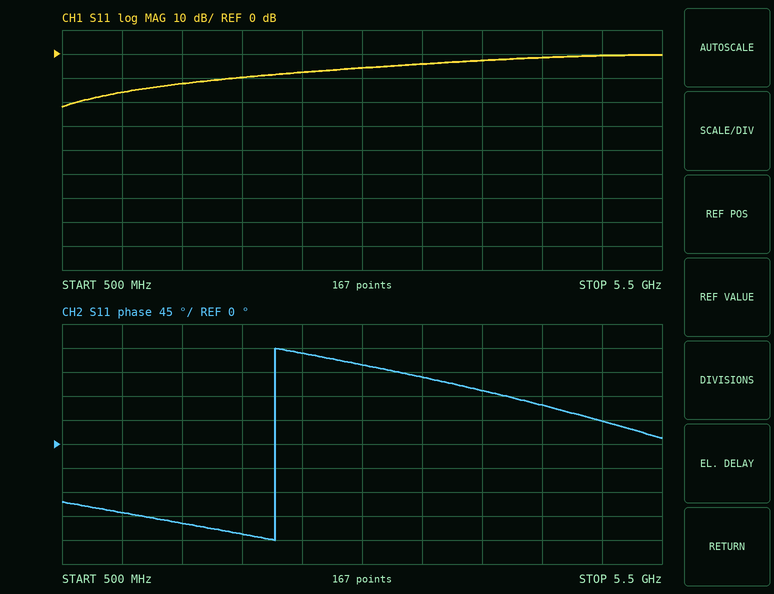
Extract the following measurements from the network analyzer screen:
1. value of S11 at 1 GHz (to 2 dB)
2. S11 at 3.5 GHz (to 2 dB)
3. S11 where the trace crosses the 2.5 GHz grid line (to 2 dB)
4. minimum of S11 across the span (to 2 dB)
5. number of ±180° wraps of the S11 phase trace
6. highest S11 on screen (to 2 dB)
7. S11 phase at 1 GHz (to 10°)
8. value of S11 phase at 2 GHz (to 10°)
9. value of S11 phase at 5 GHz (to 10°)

-16 dB
-4 dB
-8 dB
-22 dB
1
0 dB
-130°
-170°
40°
